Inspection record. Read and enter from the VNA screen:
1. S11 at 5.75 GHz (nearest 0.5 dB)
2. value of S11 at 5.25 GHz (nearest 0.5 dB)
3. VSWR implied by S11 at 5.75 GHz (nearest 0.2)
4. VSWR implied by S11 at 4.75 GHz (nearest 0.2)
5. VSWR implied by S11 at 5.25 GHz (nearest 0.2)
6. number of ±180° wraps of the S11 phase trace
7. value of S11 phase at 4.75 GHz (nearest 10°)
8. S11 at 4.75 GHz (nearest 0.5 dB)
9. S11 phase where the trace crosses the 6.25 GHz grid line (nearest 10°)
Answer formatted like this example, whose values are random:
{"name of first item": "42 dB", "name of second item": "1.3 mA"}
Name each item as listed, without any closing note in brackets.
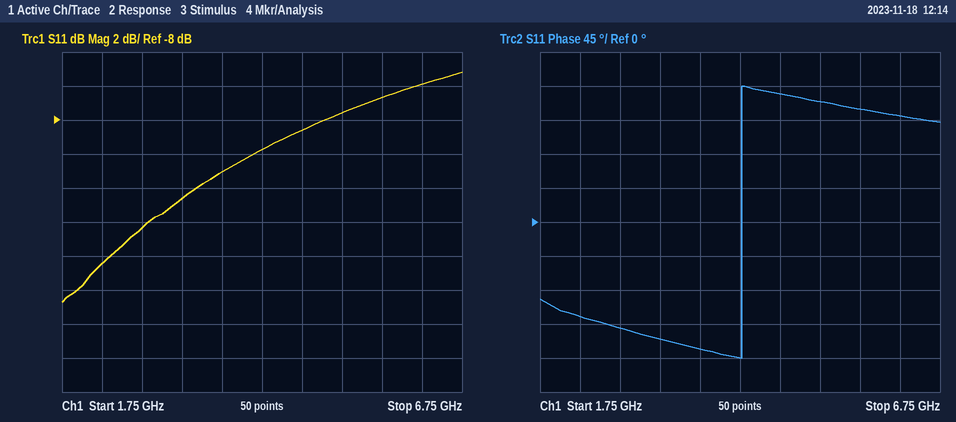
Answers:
{"S11 at 5.75 GHz": "-6.5 dB", "value of S11 at 5.25 GHz": "-7.5 dB", "VSWR implied by S11 at 5.75 GHz": "2.8", "VSWR implied by S11 at 4.75 GHz": "2.2", "VSWR implied by S11 at 5.25 GHz": "2.4", "number of ±180° wraps of the S11 phase trace": "1", "value of S11 phase at 4.75 GHz": "170°", "S11 at 4.75 GHz": "-8.5 dB", "S11 phase where the trace crosses the 6.25 GHz grid line": "140°"}
